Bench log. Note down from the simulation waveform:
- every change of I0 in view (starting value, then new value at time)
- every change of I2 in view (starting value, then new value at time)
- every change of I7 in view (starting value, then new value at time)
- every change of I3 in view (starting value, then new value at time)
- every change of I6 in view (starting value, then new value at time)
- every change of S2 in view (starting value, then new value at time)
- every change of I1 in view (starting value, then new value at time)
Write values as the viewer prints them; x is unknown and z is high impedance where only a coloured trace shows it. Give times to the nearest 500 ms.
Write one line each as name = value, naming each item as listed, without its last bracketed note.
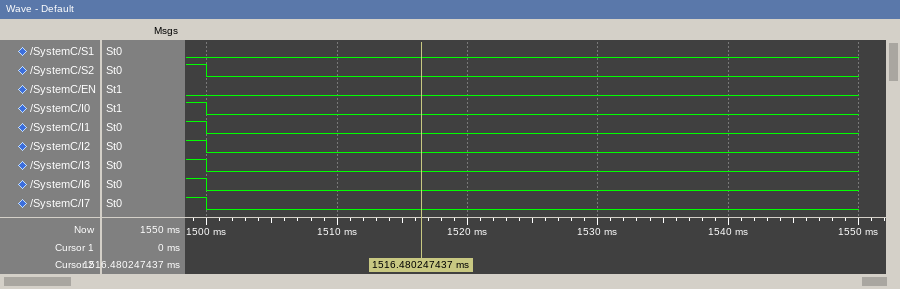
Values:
every change of I0 in view = 1, 0 at 1500 ms
every change of I2 in view = 1, 0 at 1500 ms
every change of I7 in view = 1, 0 at 1500 ms
every change of I3 in view = 1, 0 at 1500 ms
every change of I6 in view = 1, 0 at 1500 ms
every change of S2 in view = 1, 0 at 1500 ms
every change of I1 in view = 1, 0 at 1500 ms
